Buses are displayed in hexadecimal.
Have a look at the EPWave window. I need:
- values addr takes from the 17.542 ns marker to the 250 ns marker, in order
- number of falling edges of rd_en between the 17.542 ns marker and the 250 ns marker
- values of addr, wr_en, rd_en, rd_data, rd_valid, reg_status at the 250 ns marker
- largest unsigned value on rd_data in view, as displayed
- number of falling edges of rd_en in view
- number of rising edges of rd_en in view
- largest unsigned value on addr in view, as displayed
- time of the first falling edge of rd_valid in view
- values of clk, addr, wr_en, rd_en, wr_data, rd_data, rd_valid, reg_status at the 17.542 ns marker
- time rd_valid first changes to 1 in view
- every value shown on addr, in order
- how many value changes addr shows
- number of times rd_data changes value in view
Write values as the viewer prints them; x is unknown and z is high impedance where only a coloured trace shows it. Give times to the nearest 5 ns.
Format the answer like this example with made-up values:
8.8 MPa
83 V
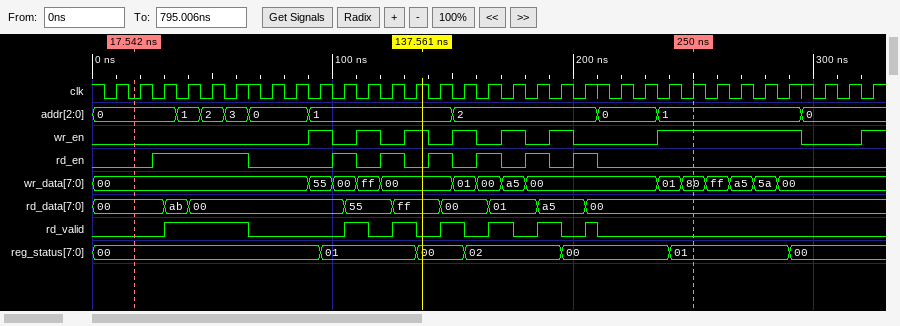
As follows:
0, 1, 2, 3, 0, 1, 2, 0, 1
7
addr=1, wr_en=1, rd_en=0, rd_data=00, rd_valid=0, reg_status=01
ff
7
7
3
65 ns
clk=0, addr=0, wr_en=0, rd_en=0, wr_data=00, rd_data=00, rd_valid=0, reg_status=00
30 ns
0, 1, 2, 3, 0, 1, 2, 0, 1, 0
9
8
